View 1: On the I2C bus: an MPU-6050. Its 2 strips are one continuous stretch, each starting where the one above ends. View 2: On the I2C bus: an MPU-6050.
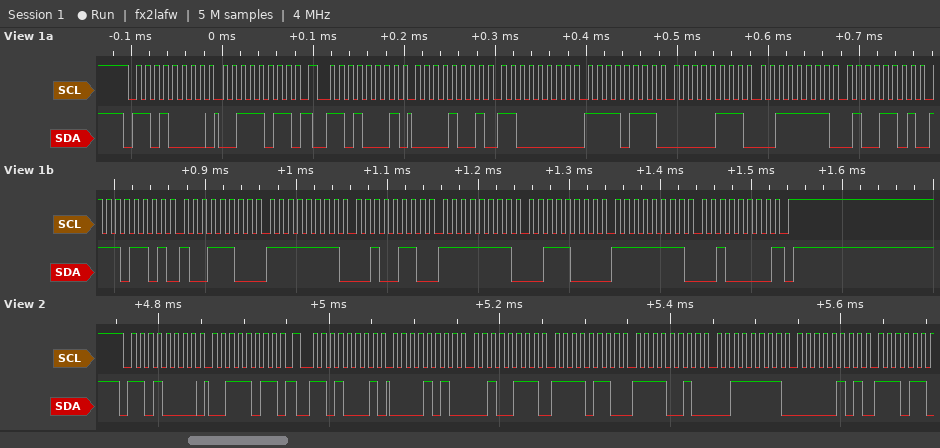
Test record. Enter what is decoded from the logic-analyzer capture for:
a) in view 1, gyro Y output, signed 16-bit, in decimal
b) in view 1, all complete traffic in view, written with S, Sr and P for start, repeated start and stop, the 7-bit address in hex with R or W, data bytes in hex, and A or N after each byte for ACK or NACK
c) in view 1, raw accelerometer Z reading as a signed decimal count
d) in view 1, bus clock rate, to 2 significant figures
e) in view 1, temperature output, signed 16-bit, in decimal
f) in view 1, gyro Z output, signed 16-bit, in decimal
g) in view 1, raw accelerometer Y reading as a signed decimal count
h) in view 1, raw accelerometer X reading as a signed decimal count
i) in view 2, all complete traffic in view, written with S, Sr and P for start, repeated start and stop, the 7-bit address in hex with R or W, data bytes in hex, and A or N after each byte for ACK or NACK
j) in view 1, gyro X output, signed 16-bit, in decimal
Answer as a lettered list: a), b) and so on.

a) -200
b) S 68W A 3B A Sr 68R A 09 A C0 A F7 A 07 A 3F A 4D A ED A 9C A FF A 26 A FF A 38 A FF A 20 N P
c) 16205
d) 100 kHz
e) -4708
f) -224
g) -2297
h) 2496
i) S 68W A 3B A Sr 68R A 0A A 27 A F6 A F2 A 3F A 05 A
j) -218
